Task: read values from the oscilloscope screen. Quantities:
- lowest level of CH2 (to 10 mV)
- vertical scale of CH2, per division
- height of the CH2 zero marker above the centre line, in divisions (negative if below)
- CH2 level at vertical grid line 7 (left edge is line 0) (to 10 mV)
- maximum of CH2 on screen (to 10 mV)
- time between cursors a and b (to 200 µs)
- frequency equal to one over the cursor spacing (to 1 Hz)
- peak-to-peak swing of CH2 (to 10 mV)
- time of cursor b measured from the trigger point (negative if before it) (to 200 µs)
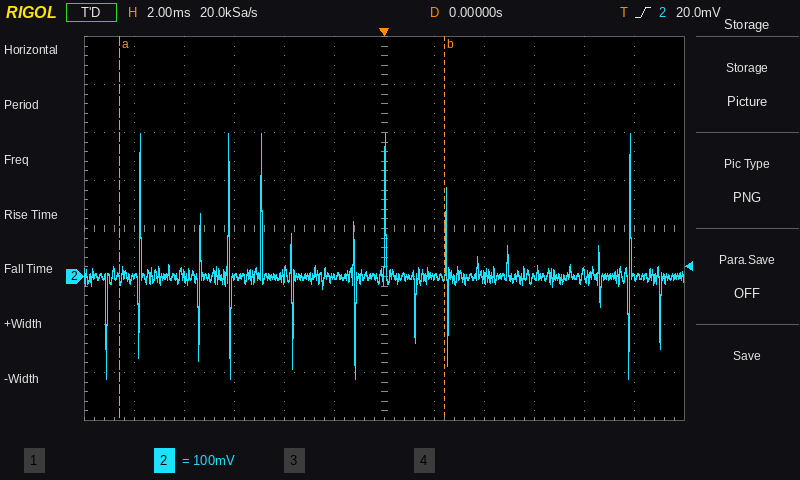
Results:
-210 mV
100 mV
-1.0 div
0 mV
300 mV
13.0 ms
77 Hz
510 mV
+2.4 ms
